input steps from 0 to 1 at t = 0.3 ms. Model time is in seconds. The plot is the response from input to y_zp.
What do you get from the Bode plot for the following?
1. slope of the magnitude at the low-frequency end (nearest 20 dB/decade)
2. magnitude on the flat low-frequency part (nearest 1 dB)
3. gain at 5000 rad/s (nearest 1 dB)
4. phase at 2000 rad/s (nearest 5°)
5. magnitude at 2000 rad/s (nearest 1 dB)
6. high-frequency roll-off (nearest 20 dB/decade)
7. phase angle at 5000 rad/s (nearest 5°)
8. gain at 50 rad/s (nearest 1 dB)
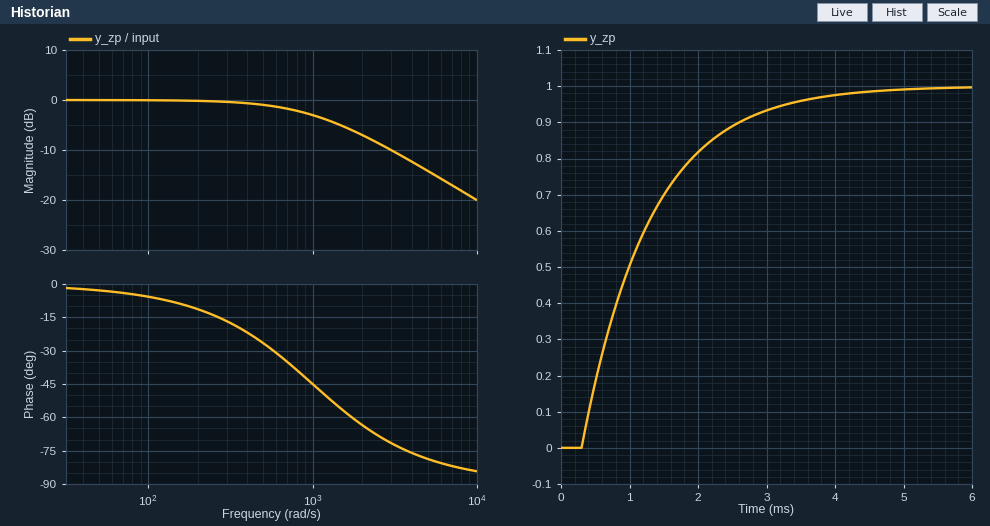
0 dB/decade
0 dB
-14 dB
-65°
-7 dB
-20 dB/decade
-80°
0 dB
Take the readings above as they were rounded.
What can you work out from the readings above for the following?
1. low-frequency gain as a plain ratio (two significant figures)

1.0
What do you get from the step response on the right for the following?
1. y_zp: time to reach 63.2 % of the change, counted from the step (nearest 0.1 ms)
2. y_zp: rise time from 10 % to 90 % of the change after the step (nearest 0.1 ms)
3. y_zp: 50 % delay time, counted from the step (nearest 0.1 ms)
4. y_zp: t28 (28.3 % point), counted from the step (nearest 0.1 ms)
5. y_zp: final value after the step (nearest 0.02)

1.0 ms
2.2 ms
0.7 ms
0.3 ms
1.00
